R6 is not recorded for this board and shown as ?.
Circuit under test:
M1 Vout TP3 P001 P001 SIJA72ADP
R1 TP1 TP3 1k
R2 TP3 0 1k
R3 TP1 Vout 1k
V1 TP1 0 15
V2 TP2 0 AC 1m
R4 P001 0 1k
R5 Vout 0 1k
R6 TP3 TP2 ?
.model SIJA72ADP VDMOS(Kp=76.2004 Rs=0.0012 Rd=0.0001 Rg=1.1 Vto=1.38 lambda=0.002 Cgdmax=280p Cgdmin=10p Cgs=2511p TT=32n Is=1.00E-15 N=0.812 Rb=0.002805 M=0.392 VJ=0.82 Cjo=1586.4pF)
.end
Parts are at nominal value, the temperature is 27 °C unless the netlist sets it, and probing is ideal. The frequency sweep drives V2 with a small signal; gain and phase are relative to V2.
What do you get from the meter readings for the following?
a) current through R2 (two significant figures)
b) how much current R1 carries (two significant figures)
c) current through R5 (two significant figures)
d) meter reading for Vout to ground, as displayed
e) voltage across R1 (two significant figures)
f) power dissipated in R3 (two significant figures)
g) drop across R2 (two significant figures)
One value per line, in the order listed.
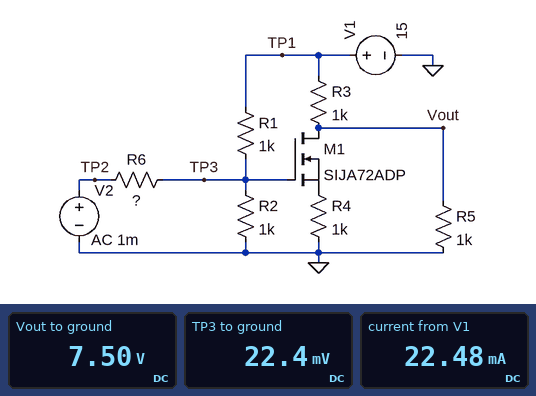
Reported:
22 µA
15 mA
7.5 mA
7.50 V
15 V
56 mW
22 mV
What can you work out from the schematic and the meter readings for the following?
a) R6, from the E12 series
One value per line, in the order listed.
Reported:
1.5 Ω
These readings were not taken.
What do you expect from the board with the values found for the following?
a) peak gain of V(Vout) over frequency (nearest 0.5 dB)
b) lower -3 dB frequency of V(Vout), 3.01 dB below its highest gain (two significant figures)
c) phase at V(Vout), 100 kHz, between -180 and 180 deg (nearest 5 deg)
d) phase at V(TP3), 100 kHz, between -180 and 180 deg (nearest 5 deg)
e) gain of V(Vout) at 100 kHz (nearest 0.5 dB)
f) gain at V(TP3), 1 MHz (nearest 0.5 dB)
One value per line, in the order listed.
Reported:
0 dB
610 kHz
105 deg
0 deg
-17.0 dB
0 dB
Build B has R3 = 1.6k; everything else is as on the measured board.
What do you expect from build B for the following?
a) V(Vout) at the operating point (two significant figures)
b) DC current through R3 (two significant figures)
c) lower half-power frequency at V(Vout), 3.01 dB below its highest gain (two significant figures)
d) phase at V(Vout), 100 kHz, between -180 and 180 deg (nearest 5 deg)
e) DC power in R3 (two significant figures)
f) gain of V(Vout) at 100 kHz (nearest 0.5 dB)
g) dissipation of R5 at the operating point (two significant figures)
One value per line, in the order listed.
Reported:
5.8 V
5.8 mA
470 kHz
100 deg
53 mW
-14.5 dB
33 mW
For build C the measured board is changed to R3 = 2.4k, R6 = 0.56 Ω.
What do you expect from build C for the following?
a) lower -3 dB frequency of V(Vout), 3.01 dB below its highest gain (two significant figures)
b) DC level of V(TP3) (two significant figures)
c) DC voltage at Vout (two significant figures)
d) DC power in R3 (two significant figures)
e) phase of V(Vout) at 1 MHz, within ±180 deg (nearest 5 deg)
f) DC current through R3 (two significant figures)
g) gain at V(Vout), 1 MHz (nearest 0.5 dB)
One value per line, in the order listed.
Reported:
380 kHz
8.4 mV
4.4 V
47 mW
25 deg
4.4 mA
-0.5 dB
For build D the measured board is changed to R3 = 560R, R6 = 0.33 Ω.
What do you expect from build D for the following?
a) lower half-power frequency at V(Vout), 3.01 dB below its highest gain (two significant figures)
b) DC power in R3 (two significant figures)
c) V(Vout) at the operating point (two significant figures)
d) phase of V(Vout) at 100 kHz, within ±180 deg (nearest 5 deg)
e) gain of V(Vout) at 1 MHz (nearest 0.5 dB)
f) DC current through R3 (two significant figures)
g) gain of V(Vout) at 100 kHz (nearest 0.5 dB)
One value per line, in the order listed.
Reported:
910 kHz
52 mW
9.6 V
110 deg
-2.5 dB
9.6 mA
-20.0 dB
